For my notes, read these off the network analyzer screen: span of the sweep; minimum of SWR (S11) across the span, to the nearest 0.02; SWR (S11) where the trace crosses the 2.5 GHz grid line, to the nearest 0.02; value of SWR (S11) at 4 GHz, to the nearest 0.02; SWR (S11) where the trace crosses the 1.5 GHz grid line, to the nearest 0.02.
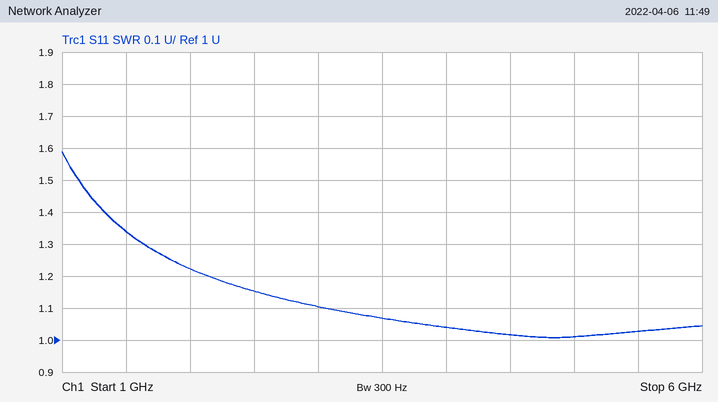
5 GHz
1.00
1.16
1.04
1.34
